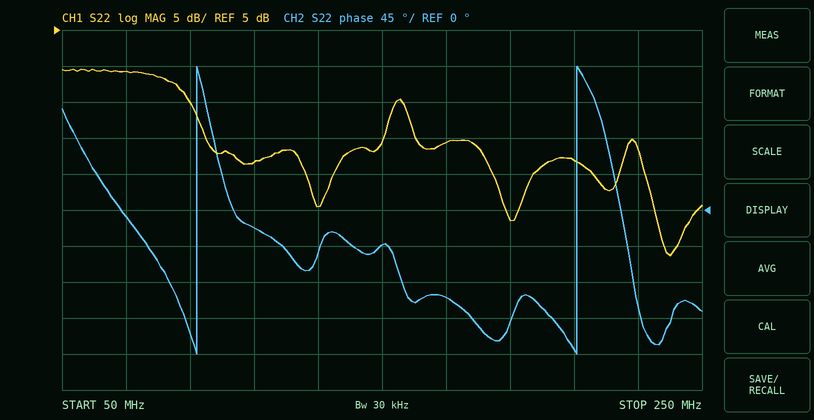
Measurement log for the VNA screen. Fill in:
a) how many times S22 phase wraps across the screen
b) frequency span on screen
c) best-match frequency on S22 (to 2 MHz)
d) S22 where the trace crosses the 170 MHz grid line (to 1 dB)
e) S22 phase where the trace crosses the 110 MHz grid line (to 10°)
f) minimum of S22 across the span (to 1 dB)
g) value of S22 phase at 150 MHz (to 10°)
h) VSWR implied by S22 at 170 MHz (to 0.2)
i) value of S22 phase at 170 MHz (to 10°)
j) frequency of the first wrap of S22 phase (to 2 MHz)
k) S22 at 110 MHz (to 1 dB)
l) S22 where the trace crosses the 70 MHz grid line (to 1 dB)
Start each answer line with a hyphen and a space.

- 2
- 200 MHz
- 240 MHz
- -11 dB
- -20°
- -26 dB
- -40°
- 1.8
- -110°
- 92 MHz
- -13 dB
- -1 dB
